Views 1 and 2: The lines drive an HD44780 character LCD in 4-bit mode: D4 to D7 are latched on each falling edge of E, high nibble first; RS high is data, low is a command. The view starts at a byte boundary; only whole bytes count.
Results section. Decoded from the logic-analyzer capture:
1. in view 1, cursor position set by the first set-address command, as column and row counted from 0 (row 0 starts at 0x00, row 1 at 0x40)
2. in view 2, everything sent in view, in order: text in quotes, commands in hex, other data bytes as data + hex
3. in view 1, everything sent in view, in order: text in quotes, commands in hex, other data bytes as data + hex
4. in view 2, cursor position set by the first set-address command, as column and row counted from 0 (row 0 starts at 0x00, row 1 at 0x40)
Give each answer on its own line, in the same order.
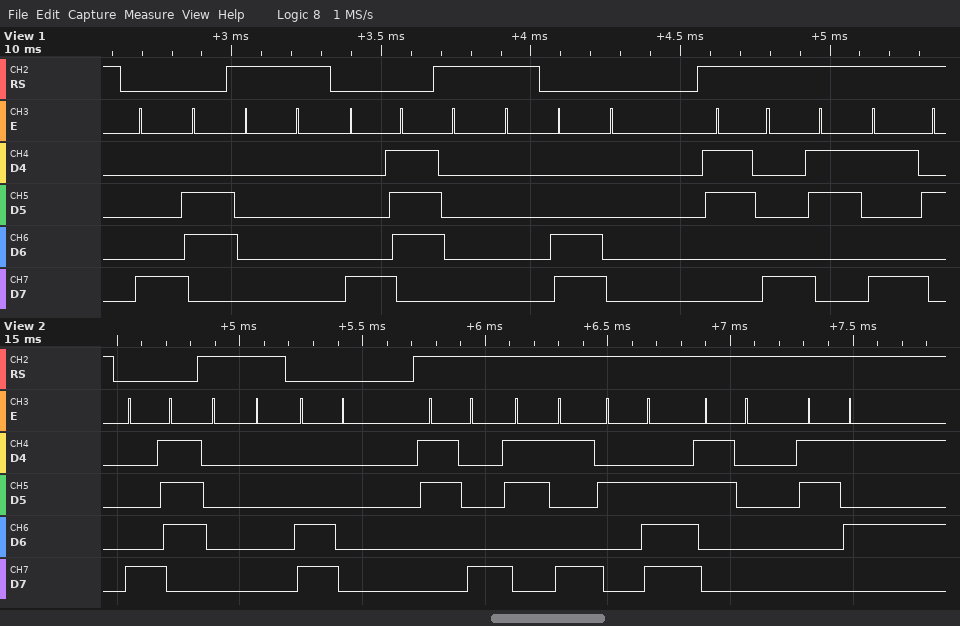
column 6, row 0
0x87 data 00 0xC0 "89.05"
0x86 data 00 0x87 data 00 0xC0 "89"
column 7, row 0
